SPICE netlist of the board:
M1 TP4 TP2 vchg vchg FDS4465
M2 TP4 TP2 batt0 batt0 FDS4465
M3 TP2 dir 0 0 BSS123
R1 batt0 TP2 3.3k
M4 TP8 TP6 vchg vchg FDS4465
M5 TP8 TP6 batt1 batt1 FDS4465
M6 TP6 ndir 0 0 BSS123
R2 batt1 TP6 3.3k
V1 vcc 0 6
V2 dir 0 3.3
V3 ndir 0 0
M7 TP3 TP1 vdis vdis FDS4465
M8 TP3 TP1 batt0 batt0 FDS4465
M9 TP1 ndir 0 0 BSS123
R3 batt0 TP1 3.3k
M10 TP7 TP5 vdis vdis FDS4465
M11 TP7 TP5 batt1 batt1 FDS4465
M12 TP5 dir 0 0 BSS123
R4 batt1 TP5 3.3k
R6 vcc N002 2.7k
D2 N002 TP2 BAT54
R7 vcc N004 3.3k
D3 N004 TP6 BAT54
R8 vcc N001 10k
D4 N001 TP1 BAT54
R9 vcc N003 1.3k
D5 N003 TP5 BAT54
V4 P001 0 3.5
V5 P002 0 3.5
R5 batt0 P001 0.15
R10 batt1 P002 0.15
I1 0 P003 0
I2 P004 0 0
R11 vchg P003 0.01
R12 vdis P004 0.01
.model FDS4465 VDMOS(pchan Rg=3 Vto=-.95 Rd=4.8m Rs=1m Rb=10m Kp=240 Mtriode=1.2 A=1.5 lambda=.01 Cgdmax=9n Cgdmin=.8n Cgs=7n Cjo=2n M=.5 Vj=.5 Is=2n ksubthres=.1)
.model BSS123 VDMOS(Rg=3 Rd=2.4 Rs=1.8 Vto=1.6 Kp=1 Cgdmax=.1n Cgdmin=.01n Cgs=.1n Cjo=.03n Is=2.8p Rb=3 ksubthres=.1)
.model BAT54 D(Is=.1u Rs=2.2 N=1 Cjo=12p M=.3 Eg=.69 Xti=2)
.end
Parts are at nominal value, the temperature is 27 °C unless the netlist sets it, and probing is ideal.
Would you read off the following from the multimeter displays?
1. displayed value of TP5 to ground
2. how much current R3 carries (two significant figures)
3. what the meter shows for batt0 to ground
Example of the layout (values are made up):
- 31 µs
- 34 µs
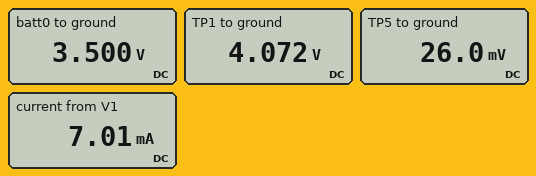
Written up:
- 26.0 mV
- 170 µA
- 3.500 V
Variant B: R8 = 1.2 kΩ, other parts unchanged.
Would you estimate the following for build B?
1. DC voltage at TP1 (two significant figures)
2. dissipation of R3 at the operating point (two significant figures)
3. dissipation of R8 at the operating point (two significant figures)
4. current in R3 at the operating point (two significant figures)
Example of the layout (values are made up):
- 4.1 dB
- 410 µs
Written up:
- 5.2 V
- 850 µW
- 310 µW
- 510 µA
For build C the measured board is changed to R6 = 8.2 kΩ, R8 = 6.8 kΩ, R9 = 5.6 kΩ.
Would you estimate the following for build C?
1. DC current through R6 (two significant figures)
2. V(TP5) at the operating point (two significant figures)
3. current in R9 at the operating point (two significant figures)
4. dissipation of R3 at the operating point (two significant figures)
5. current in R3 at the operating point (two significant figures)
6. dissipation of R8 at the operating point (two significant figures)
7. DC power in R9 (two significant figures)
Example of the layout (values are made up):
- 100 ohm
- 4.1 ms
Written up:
- 700 µA
- 10 mV
- 1.0 mA
- 170 µW
- 230 µA
- 350 µW
- 5.9 mW
